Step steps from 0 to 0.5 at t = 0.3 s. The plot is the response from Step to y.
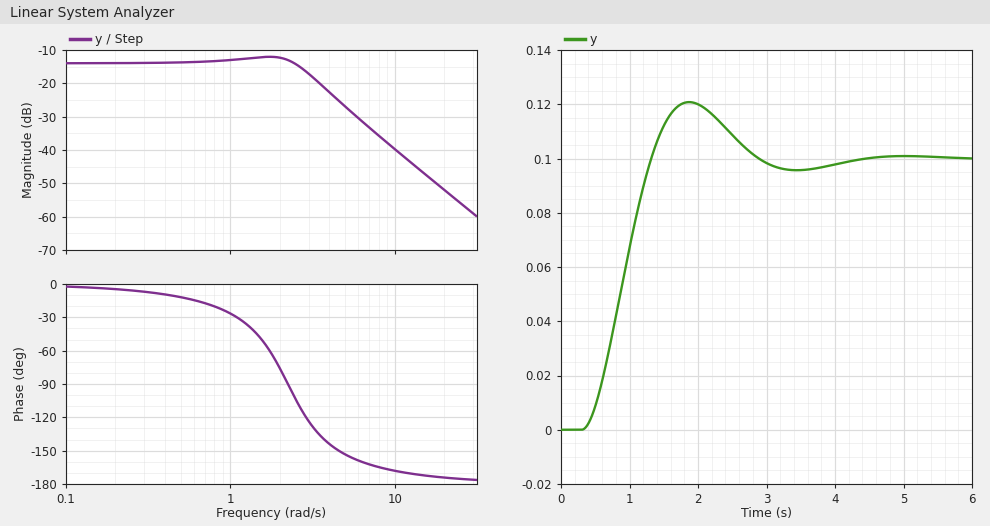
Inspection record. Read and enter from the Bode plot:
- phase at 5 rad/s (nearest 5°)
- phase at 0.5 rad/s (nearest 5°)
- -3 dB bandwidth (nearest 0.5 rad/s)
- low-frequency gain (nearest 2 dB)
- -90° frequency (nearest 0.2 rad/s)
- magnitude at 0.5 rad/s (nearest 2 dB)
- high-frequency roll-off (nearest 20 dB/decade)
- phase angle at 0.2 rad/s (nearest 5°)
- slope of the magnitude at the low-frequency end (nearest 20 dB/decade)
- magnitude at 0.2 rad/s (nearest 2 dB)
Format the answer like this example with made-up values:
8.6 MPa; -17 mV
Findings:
-155°; -10°; 3.0 rad/s; -14 dB; 2.2 rad/s; -14 dB; -40 dB/decade; -5°; 0 dB/decade; -14 dB
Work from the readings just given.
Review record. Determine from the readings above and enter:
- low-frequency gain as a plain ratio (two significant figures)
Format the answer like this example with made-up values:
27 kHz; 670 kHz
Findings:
0.20
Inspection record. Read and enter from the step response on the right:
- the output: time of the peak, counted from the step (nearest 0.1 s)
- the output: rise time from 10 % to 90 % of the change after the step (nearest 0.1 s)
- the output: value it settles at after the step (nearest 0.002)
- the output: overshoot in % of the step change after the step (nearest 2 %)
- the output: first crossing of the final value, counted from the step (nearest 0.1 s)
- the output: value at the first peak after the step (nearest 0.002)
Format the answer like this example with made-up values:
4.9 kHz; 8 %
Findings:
1.6 s; 0.7 s; 0.100; 20 %; 1.0 s; 0.120
